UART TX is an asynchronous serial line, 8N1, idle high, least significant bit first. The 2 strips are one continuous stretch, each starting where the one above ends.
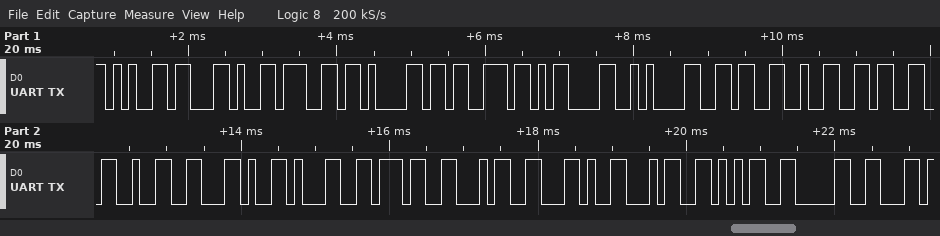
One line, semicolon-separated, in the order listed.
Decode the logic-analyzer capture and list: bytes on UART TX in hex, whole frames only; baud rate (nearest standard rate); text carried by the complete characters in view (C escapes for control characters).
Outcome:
65 2C 67 61 73 0D 0A 36 32 33 32 2C 31 37 34 2C 34 35 30; 9600 baud; "e,gas\r\n6232,174,450"
